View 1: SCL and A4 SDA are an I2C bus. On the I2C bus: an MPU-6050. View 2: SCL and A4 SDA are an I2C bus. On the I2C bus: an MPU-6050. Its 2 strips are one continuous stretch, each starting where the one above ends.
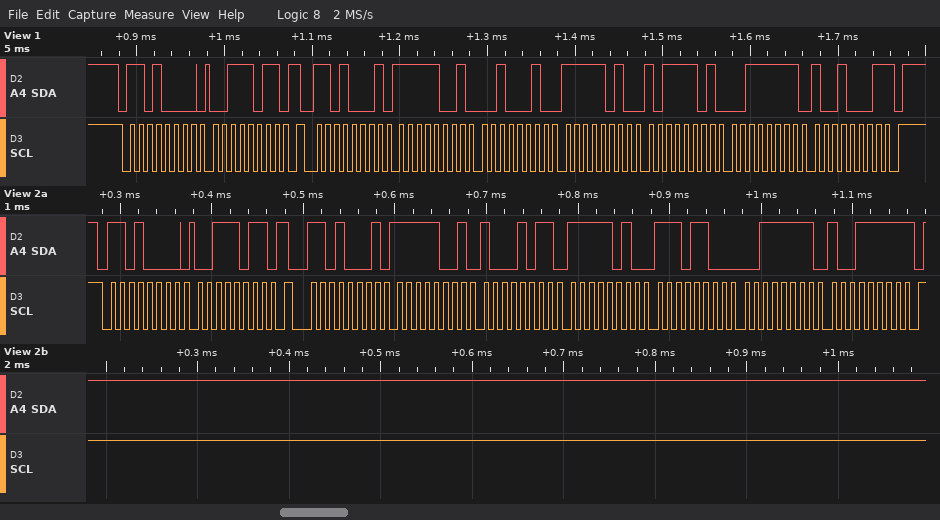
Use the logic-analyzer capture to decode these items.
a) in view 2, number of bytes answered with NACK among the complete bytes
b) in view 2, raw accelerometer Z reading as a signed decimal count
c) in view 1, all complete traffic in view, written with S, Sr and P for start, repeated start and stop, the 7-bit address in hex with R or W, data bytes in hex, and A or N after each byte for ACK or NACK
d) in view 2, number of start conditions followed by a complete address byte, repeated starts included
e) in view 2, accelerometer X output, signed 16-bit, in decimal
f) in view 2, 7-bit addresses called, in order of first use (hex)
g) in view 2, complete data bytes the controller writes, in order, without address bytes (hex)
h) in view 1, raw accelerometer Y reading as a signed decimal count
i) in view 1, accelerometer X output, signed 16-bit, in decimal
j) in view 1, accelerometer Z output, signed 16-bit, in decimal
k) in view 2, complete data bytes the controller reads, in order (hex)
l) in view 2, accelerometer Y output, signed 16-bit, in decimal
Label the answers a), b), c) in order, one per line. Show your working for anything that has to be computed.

a) 1
b) 0x3F9F = 16287
c) S 68W A 3B A Sr 68R A F9 A 22 A FA A BD A 3F A 91 N P
d) 2
e) 0xF98B = -1653
f) 0x68
g) 3B
h) 0xFABD = -1347
i) 0xF922 = -1758
j) 0x3F91 = 16273
k) F9 8B FA EC 3F 9F
l) 0xFAEC = -1300
